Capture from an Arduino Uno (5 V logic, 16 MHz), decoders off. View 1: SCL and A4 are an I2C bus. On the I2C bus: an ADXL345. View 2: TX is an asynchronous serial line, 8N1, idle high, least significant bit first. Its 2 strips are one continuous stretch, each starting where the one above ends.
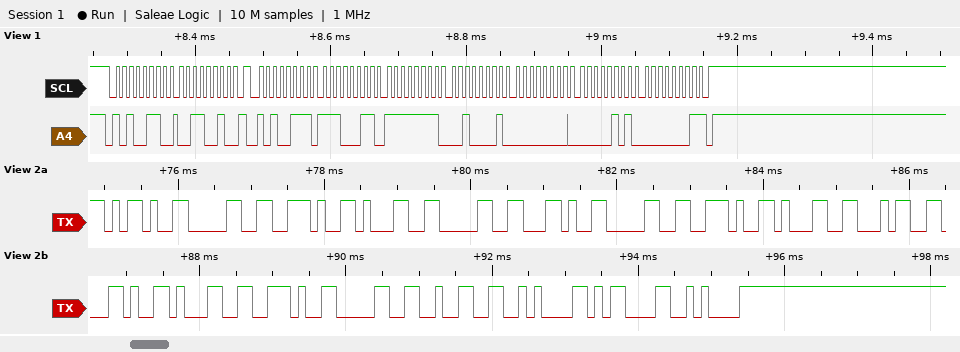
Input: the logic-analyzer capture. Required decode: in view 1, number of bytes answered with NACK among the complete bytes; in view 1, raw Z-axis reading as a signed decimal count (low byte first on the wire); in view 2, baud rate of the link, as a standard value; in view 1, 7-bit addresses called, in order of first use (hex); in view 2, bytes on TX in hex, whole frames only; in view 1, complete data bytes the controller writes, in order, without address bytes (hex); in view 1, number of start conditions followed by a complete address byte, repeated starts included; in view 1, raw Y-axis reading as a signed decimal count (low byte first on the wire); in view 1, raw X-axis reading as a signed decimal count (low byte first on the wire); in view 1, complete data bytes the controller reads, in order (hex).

1
261
9600 baud
0x53
2D 30 2E 31 30 2C 30 2E 31 34 2C 31 2E 30 32 0A 0D 0A
32
2
33
-29
E3 FF 21 00 05 01
